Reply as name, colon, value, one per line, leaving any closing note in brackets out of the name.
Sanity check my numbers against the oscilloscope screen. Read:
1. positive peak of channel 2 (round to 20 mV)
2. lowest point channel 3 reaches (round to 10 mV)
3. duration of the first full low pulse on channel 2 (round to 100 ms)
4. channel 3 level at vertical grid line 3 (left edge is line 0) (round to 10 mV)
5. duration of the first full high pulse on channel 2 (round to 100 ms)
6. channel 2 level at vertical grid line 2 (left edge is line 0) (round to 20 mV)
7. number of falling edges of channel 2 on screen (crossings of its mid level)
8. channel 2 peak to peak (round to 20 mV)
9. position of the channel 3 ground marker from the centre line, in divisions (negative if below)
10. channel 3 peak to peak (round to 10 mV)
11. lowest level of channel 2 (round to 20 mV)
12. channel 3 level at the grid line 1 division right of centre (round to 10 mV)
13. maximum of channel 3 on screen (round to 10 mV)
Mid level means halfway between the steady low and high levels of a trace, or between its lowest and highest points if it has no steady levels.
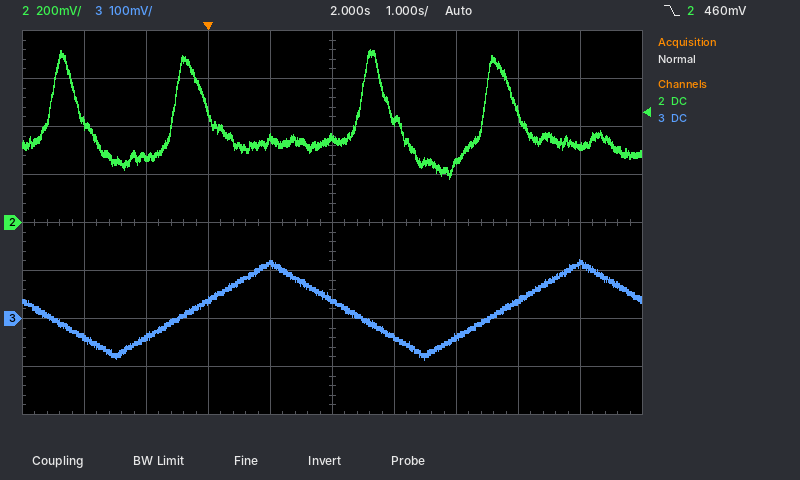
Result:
positive peak of channel 2: 720 mV
lowest point channel 3 reaches: -90 mV
duration of the first full low pulse on channel 2: 1.5 s
channel 3 level at vertical grid line 3 (left edge is line 0): 40 mV
duration of the first full high pulse on channel 2: 500 ms
channel 2 level at vertical grid line 2 (left edge is line 0): 280 mV
number of falling edges of channel 2 on screen: 4
channel 2 peak to peak: 540 mV
position of the channel 3 ground marker from the centre line, in divisions: -2.0 div
channel 3 peak to peak: 210 mV
lowest level of channel 2: 180 mV
channel 3 level at the grid line 1 division right of centre: -40 mV
maximum of channel 3 on screen: 120 mV
